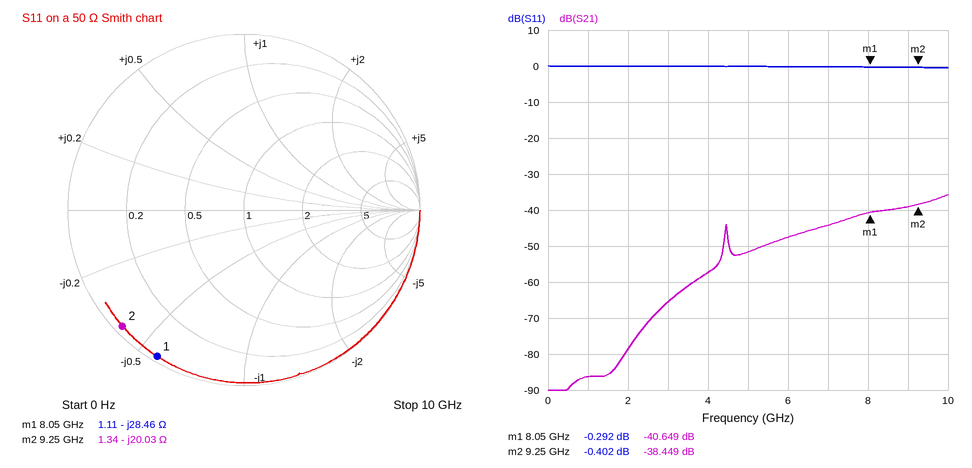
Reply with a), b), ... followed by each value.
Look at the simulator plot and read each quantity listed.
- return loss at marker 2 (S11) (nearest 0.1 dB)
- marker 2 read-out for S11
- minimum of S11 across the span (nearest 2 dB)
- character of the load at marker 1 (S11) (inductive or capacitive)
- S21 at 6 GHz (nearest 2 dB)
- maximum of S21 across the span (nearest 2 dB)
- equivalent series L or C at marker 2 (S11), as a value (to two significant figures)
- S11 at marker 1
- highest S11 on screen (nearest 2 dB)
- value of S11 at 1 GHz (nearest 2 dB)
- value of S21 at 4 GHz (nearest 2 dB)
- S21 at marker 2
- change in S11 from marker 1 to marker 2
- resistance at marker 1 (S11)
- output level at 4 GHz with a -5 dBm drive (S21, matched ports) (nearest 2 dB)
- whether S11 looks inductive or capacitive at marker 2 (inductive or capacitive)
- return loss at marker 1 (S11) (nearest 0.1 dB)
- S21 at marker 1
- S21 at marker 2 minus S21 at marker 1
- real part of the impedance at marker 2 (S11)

a) 0.4 dB
b) -0.402 dB
c) 0 dB
d) capacitive
e) -48 dB
f) -36 dB
g) 860 fF
h) -0.292 dB
i) 0 dB
j) 0 dB
k) -58 dB
l) -38.449 dB
m) -0.110 dB
n) 1.11 Ω
o) -62 dBm
p) capacitive
q) 0.3 dB
r) -40.649 dB
s) 2.200 dB
t) 1.34 Ω
